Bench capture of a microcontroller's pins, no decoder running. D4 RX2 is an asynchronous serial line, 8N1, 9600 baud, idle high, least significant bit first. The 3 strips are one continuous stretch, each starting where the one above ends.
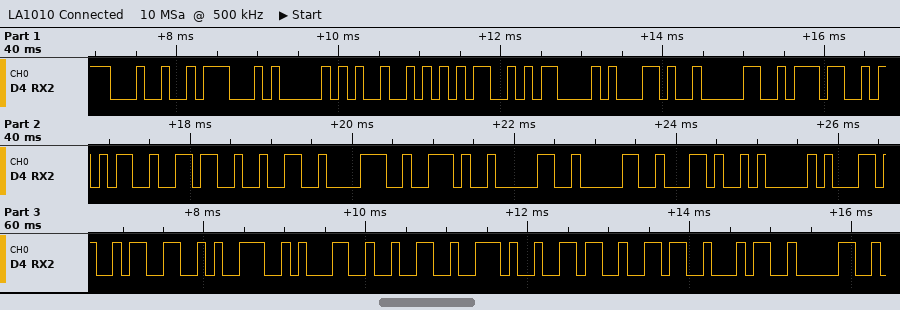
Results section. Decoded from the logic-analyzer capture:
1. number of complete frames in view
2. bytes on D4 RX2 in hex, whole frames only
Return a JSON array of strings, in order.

["28", "24 47 50 52 4D 43 2C 30 37 35 36 32 38 2E 30 30 2C 41 2C 33 39 31 32 2E 36 36 34 30"]
